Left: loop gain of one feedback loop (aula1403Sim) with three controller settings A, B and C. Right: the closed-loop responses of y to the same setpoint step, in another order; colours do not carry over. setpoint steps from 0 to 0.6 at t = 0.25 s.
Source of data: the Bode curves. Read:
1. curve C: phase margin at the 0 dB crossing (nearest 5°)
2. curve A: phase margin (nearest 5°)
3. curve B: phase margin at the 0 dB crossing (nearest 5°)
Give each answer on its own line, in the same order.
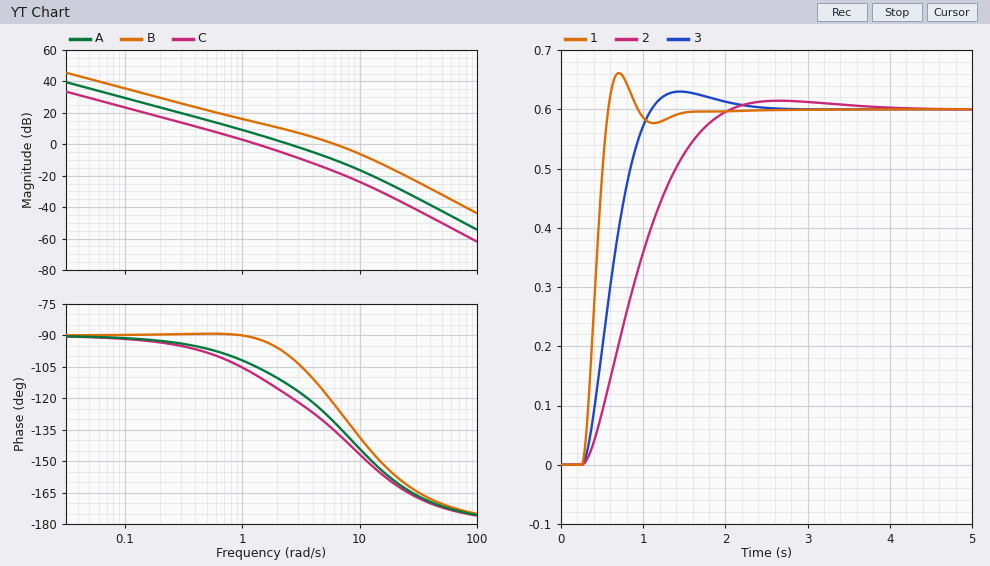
70°
65°
55°
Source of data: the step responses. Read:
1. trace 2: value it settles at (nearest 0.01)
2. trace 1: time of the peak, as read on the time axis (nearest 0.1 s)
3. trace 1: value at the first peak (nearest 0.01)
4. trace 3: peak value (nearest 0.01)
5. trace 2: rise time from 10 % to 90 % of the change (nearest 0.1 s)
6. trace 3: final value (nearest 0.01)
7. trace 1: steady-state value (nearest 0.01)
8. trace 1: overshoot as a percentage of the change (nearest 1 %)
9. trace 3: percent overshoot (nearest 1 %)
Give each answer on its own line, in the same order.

0.60
0.7 s
0.66
0.63
1.1 s
0.60
0.60
10 %
5 %
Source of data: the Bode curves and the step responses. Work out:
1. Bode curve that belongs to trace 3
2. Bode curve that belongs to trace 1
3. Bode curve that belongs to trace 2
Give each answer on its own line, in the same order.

A
B
C
